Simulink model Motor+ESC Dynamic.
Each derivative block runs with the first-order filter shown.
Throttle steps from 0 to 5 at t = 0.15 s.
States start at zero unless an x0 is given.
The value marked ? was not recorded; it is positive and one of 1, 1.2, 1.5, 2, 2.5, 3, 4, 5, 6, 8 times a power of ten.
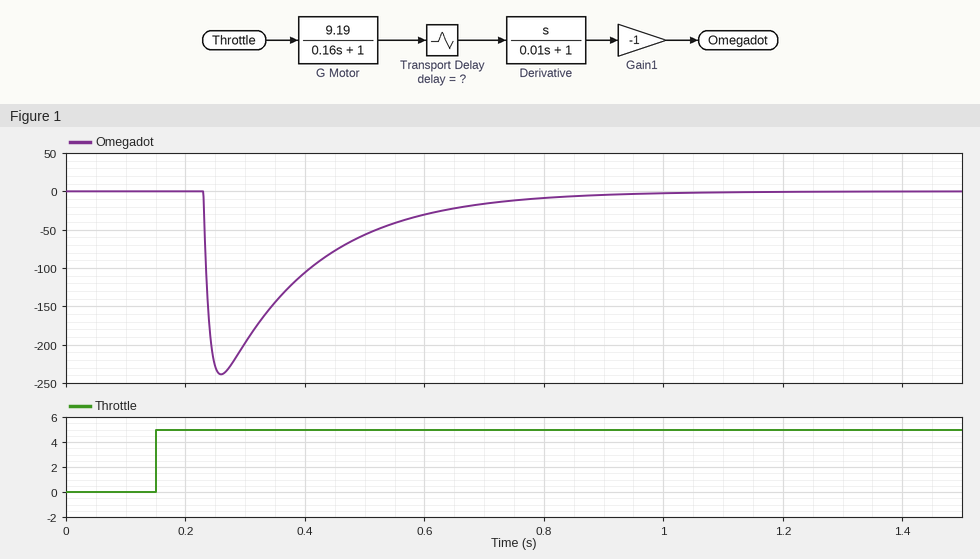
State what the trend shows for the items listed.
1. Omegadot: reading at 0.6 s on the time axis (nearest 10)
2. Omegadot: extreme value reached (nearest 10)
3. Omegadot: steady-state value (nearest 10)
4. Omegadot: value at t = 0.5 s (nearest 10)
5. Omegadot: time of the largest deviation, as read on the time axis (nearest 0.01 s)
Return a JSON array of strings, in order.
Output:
["-30", "-240", "0", "-60", "0.26 s"]
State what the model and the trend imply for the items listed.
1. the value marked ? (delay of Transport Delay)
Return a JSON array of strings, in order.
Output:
["0.08"]
